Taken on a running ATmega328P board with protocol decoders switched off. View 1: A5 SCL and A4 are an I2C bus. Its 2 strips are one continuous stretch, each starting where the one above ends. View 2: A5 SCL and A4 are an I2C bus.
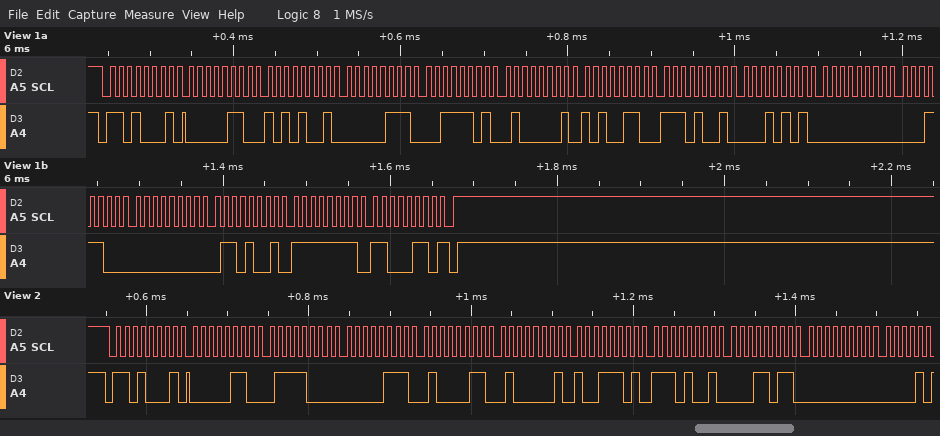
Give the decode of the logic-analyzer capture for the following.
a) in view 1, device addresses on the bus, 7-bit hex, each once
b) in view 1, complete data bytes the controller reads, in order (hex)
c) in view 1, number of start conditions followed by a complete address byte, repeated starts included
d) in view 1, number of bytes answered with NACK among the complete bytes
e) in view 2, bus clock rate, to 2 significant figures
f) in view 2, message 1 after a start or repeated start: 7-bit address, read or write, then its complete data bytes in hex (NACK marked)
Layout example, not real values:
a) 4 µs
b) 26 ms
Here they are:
a) 0x68
b) 06 A9 07 3D 41 A6 E9 15 00 1C 00 69 FF C6
c) 1
d) 1
e) 100 kHz
f) 0x68 read: 06 78 07 43 41 9D E9 1B 00
